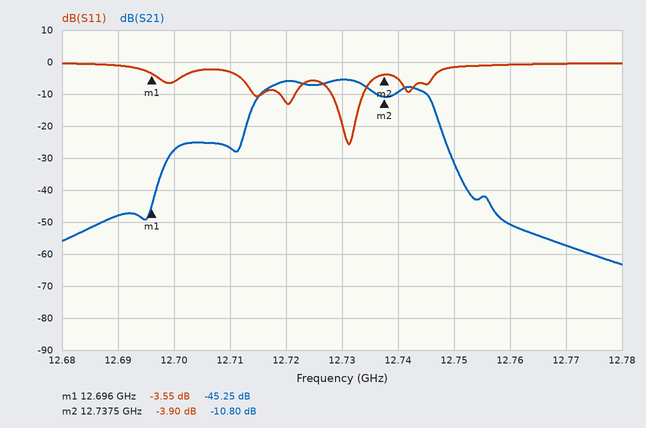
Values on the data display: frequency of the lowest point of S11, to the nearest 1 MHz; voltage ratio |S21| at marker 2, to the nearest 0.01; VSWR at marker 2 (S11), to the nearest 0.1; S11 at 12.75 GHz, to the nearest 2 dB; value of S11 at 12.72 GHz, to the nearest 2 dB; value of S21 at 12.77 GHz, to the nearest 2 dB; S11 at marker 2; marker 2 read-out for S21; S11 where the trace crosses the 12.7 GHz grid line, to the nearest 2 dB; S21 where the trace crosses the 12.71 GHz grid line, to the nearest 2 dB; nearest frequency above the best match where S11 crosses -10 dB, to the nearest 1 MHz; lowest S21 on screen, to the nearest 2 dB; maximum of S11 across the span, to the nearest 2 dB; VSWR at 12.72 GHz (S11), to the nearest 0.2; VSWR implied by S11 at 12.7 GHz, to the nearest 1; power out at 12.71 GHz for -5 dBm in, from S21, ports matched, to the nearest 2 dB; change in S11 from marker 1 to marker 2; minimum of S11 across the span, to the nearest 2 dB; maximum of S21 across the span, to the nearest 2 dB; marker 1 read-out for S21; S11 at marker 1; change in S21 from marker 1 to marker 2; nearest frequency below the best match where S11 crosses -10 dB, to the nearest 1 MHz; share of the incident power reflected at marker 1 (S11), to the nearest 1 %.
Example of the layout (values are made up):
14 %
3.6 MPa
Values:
12.731 GHz
0.29
4.5
-2 dB
-12 dB
-58 dB
-3.90 dB
-10.80 dB
-6 dB
-26 dB
12.734 GHz
-64 dB
0 dB
1.6
3
-32 dBm
-0.35 dB
-26 dB
-6 dB
-45.25 dB
-3.55 dB
34.45 dB
12.728 GHz
44 %
